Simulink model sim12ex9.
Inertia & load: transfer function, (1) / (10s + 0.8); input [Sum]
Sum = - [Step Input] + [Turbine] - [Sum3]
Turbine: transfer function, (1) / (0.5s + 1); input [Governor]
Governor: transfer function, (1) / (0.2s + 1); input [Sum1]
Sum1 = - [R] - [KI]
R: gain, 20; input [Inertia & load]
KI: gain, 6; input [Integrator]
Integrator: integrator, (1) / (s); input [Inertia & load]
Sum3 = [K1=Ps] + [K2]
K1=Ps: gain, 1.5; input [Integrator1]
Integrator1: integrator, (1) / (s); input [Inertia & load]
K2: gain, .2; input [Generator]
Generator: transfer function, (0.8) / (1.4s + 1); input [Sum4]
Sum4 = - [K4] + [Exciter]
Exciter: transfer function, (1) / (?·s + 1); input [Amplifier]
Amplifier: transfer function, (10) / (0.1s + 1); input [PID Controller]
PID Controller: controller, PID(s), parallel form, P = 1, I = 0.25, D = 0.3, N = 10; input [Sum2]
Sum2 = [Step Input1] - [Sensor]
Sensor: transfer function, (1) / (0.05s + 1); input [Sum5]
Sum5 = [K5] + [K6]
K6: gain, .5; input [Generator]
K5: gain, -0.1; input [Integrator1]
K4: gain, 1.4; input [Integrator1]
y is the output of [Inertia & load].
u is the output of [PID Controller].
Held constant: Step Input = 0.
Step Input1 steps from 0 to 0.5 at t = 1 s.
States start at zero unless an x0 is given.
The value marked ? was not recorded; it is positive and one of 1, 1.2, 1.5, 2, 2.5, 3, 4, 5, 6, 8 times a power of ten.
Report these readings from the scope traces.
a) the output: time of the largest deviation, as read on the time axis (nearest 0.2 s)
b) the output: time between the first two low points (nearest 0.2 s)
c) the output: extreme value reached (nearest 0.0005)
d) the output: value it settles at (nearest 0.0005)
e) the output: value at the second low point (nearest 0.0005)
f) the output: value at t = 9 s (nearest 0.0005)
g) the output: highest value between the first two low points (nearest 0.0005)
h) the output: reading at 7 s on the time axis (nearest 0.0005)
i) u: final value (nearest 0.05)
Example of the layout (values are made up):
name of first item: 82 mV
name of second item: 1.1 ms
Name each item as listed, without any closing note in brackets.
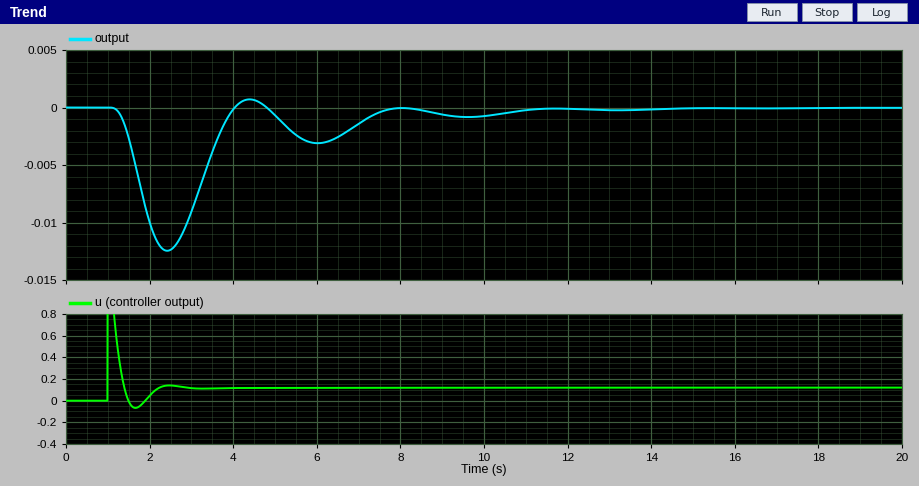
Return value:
the output: time of the largest deviation, as read on the time axis: 2.4 s
the output: time between the first two low points: 3.6 s
the output: extreme value reached: -0.0125
the output: value it settles at: 0.0000
the output: value at the second low point: -0.0030
the output: value at t = 9 s: -0.0005
the output: highest value between the first two low points: 0.0005
the output: reading at 7 s on the time axis: -0.0015
u: final value: 0.10
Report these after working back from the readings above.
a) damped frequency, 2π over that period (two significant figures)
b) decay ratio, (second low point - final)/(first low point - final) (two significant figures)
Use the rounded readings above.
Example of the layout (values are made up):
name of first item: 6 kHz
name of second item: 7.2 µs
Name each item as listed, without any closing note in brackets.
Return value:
damped frequency, 2π over that period: 1.7 rad/s
decay ratio, (second low point - final)/(first low point - final): 0.24
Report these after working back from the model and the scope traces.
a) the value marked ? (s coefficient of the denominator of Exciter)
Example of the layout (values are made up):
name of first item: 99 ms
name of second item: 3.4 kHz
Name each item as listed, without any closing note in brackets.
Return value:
the value marked ?: 0.4
